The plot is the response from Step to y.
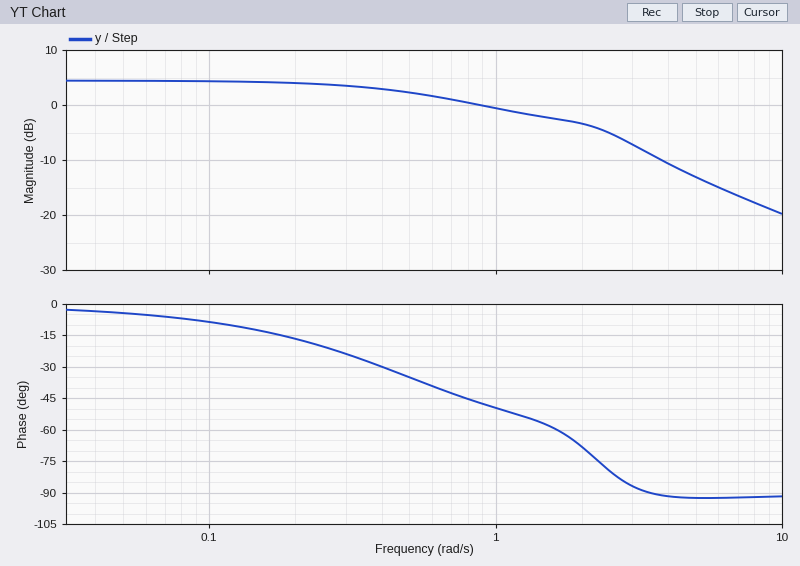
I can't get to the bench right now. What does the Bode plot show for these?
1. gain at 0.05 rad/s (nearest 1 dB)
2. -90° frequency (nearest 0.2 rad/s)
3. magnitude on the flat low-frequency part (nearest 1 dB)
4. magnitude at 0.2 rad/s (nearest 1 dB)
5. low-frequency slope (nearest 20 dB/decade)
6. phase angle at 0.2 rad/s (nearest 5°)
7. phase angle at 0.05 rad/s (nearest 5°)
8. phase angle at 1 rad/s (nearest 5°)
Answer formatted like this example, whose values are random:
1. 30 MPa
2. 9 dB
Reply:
1. 4 dB
2. 3.4 rad/s
3. 4 dB
4. 4 dB
5. 0 dB/decade
6. -15°
7. -5°
8. -50°
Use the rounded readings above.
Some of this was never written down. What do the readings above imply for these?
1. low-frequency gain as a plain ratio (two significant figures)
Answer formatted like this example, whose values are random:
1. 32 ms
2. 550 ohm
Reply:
1. 1.6
